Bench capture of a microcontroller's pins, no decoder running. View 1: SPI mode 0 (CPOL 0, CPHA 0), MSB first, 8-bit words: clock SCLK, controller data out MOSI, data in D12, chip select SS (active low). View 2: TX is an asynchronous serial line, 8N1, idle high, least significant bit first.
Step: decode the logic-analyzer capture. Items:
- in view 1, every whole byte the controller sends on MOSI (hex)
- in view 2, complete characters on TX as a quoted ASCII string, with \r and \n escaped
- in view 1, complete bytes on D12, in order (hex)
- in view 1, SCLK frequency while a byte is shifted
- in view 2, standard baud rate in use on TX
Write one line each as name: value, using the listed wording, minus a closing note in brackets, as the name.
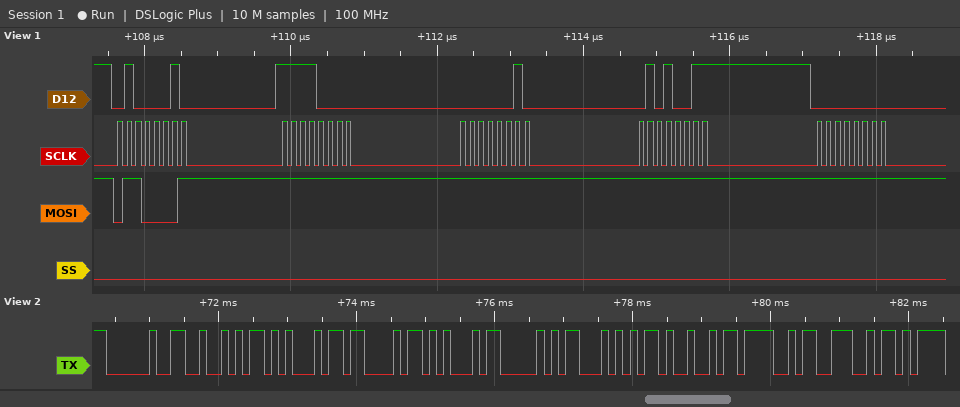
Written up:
in view 1, every whole byte the controller sends on MOSI: 61 FF FF FF FF
in view 2, complete characters on TX as a quoted ASCII string, with \r and \n escaped: " RECEPTION"
in view 1, complete bytes on D12, in order: 42 F0 02 53 00
in view 1, SCLK frequency while a byte is shifted: 8 MHz
in view 2, standard baud rate in use on TX: 9600 baud
